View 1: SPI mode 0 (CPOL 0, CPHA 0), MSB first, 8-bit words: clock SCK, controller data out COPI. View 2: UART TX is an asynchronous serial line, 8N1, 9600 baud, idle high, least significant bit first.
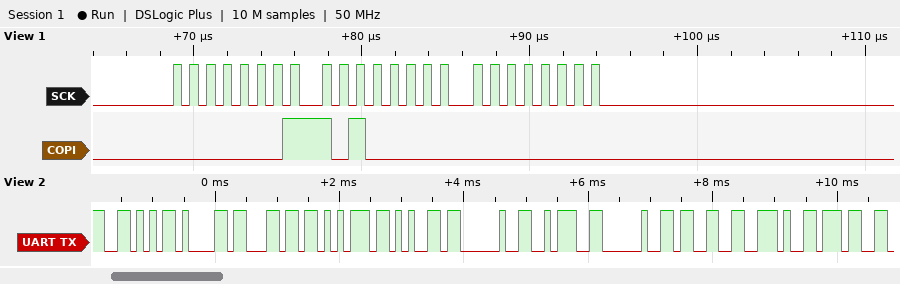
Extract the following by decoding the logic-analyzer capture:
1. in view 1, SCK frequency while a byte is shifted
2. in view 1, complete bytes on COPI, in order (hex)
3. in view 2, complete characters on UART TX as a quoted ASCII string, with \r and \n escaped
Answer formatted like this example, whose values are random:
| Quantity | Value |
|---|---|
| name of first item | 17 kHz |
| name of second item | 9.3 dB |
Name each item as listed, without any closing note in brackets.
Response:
| Quantity | Value |
|---|---|
| in view 1, SCK frequency while a byte is shifted | 1 MHz |
| in view 1, complete bytes on COPI, in order | 01 A0 00 |
| in view 2, complete characters on UART TX as a quoted ASCII string, with \r and \n escaped | "Value : 3.7" |
